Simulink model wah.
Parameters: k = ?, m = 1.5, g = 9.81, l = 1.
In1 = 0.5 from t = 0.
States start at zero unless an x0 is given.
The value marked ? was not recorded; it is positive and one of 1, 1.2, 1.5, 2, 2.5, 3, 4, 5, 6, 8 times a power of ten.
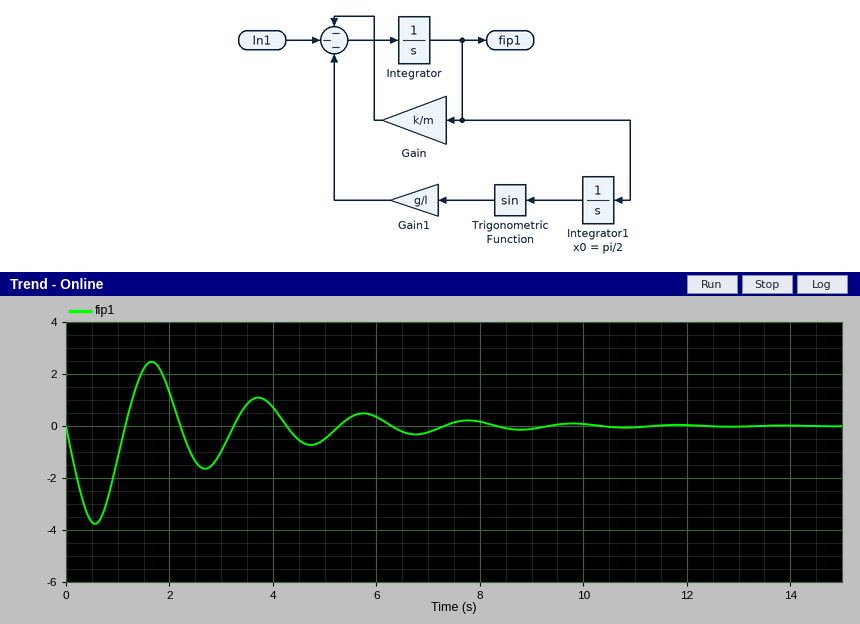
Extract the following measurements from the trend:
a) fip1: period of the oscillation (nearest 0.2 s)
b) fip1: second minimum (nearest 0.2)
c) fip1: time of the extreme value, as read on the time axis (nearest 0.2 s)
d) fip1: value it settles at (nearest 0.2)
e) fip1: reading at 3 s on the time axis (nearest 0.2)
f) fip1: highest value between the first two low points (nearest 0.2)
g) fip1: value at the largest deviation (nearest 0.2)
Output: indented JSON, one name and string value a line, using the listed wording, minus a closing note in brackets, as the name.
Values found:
{
  "fip1: period of the oscillation": "2.2 s",
  "fip1: second minimum": "-1.6",
  "fip1: time of the extreme value, as read on the time axis": "0.6 s",
  "fip1: value it settles at": "0.0",
  "fip1: reading at 3 s on the time axis": "-1.0",
  "fip1: highest value between the first two low points": "2.4",
  "fip1: value at the largest deviation": "-3.8"
}
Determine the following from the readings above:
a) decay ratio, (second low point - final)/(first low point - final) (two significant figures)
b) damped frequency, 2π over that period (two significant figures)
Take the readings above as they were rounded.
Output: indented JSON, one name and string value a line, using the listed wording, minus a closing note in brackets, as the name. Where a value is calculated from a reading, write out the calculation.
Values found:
{
  "decay ratio, (second low point - final)/(first low point - final)": "(-1.6 - 0) / (-3.8 - 0) = 0.42",
  "damped frequency, 2π over that period": "2π / 2.2 = 2.9 rad/s"
}
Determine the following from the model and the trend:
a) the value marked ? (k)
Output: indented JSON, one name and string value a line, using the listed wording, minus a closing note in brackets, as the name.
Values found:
{
  "the value marked ?": "1.2"
}
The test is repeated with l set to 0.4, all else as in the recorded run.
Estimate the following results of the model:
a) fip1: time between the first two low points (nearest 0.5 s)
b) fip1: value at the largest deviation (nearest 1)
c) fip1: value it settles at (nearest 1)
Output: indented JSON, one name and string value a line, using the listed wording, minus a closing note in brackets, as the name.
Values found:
{
  "fip1: time between the first two low points": "1.5 s",
  "fip1: value at the largest deviation": "-6",
  "fip1: value it settles at": "0"
}
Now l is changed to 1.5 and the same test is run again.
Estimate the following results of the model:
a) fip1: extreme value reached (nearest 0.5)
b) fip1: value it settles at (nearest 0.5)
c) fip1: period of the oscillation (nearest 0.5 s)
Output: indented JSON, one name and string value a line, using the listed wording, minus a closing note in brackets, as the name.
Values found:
{
  "fip1: extreme value reached": "-3.0",
  "fip1: value it settles at": "0.0",
  "fip1: period of the oscillation": "2.5 s"
}
